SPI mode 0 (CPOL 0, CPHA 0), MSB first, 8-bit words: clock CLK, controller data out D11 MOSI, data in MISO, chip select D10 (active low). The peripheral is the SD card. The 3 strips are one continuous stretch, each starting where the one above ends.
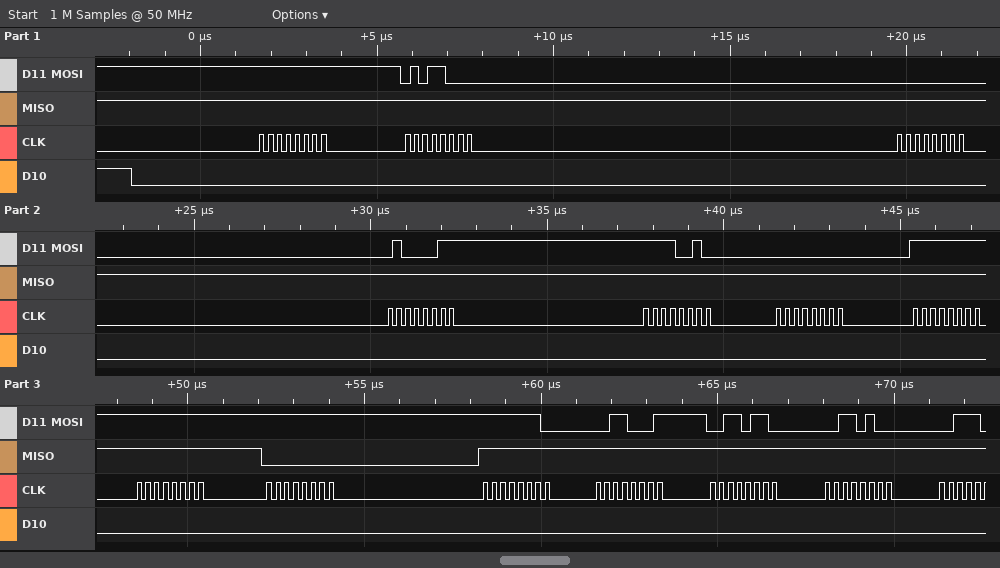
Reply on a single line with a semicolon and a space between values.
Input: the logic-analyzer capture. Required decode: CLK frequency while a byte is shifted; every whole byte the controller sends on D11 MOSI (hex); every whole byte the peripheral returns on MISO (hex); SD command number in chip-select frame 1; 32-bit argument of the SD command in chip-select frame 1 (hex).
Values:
4 MHz; 0xFF 0x58 0x00 0x43 0xF2 0x00 0xFF 0xFF 0xFF 0xFE 0x31 0x36 0x34; 0xFF 0xFF 0xFF 0xFF 0xFF 0xFF 0xFF 0xFF 0x00 0xFF 0xFF 0xFF 0xFF; CMD24; 0x0043F200
